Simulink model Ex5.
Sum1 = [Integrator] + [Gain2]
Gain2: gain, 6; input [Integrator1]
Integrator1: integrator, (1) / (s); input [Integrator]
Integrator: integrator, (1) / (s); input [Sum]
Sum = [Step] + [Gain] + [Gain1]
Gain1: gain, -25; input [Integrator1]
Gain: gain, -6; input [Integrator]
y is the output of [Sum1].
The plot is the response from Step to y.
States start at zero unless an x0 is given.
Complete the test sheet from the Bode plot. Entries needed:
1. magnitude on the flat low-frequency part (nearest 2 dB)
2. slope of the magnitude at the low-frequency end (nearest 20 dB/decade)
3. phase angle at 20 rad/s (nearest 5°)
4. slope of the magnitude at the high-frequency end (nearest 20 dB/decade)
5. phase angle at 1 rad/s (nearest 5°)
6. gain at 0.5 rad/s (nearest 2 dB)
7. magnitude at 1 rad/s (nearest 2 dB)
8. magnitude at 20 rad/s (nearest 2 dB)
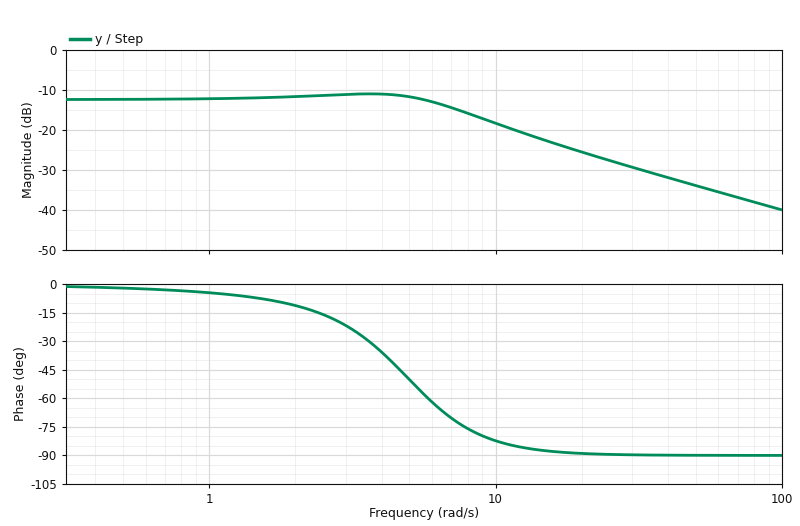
-12 dB
0 dB/decade
-90°
-20 dB/decade
-5°
-12 dB
-12 dB
-26 dB
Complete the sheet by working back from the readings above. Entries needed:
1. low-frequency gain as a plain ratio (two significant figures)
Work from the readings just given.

0.25
